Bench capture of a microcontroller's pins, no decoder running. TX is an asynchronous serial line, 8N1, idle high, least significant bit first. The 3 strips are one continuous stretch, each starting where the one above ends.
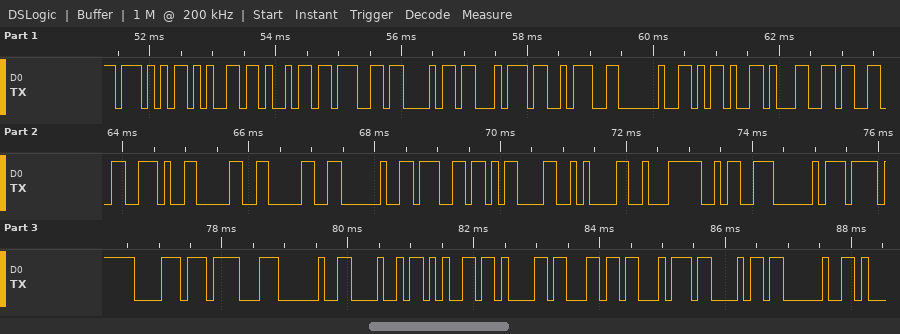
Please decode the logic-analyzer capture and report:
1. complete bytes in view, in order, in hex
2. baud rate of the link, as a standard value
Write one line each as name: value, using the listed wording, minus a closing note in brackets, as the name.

complete bytes in view, in order, in hex: 57 65 69 67 68 74 3A 20 2D 31 33 2E 30 30 20 67 0D 0A E2 9A A0 EF B8 8F 20 48 65 61 6C 74 68 20
baud rate of the link, as a standard value: 9600 baud
